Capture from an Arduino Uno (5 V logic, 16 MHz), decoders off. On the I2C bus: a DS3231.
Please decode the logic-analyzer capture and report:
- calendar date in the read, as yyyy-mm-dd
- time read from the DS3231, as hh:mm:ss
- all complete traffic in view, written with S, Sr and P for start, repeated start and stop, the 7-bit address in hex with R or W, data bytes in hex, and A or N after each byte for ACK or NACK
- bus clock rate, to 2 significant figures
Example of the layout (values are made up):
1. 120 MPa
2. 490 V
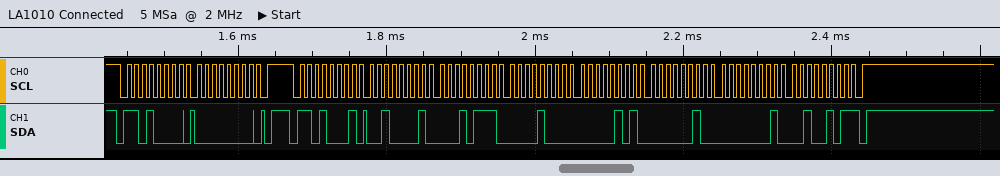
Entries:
1. 2025-01-02
2. 08:17:21
3. S 68W A 00 A P S 68R A 21 A 17 A 08 A 05 A 02 A 01 A 25 N P
4. 100 kHz
